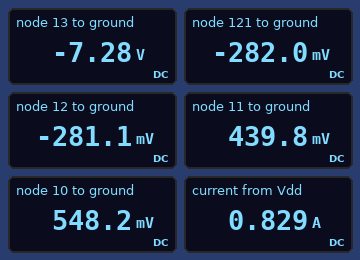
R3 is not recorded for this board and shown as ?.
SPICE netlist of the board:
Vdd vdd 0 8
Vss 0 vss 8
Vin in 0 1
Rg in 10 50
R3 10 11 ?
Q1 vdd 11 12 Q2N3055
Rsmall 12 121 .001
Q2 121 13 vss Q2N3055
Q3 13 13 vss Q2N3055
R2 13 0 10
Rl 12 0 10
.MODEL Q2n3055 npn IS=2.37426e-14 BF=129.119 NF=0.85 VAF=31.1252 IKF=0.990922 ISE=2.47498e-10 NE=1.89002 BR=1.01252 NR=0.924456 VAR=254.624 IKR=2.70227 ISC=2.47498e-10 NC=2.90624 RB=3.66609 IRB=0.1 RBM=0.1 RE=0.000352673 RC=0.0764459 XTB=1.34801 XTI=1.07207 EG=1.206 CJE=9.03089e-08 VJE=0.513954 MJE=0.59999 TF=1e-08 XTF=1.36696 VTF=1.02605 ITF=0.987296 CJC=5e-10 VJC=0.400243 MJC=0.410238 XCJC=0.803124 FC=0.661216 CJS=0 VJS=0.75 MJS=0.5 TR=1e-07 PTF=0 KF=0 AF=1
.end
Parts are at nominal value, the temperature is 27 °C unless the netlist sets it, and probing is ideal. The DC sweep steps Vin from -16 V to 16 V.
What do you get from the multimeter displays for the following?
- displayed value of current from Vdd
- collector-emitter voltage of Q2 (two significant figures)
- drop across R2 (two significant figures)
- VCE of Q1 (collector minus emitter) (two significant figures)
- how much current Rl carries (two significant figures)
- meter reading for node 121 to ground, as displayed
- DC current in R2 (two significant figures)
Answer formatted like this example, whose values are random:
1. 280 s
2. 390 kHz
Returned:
1. 0.829 A
2. 7.7 V
3. 7.3 V
4. 8.3 V
5. 28 mA
6. -282.0 mV
7. 730 mA
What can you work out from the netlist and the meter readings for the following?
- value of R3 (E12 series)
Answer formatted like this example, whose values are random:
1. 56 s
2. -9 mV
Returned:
1. 12 Ω
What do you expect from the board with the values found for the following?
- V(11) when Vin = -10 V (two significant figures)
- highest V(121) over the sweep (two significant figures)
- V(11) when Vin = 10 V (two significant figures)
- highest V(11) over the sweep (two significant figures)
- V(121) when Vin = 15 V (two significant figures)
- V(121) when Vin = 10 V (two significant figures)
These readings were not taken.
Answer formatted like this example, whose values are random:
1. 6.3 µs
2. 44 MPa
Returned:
1. -10 V
2. 7.8 V
3. 7.8 V
4. 8.8 V
5. 7.8 V
6. 7.0 V
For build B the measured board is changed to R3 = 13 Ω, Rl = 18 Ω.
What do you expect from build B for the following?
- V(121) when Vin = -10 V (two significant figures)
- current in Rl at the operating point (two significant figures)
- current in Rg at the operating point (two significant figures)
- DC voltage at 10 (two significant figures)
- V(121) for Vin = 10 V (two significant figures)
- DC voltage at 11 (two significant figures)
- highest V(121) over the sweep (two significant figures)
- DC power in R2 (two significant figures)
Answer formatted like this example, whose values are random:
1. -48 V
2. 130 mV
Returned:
1. -7.9 V
2. 17 mA
3. 9.2 mA
4. 540 mV
5. 7.4 V
6. 420 mV
7. 7.9 V
8. 5.3 W
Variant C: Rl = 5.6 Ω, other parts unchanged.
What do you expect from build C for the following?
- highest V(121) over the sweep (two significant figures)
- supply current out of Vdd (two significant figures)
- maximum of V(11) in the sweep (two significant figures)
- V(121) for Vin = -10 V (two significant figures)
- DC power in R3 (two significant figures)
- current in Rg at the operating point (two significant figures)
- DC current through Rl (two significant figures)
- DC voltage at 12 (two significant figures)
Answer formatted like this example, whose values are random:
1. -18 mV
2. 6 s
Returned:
1. 7.8 V
2. 810 mA
3. 8.7 V
4. -4.3 V
5. 920 µW
6. 8.8 mA
7. 47 mA
8. -260 mV
